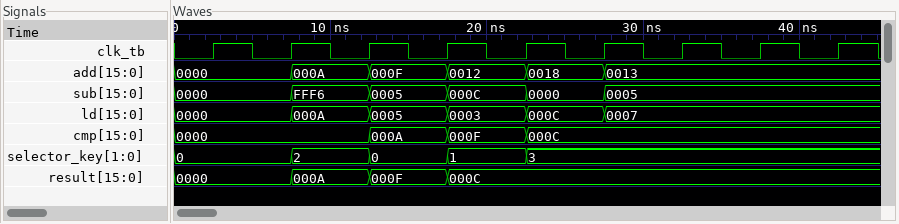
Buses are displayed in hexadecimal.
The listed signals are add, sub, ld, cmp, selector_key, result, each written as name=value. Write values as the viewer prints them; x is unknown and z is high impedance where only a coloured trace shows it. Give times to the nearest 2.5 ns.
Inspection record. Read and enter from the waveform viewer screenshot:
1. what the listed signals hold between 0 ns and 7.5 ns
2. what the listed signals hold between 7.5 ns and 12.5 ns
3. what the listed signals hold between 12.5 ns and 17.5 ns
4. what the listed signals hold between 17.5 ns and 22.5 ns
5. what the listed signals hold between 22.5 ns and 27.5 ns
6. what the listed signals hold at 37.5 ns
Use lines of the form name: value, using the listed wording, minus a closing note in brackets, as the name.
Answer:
what the listed signals hold between 0 ns and 7.5 ns: add=0000, sub=0000, ld=0000, cmp=0000, selector_key=0, result=0000
what the listed signals hold between 7.5 ns and 12.5 ns: add=000A, sub=FFF6, ld=000A, cmp=0000, selector_key=2, result=000A
what the listed signals hold between 12.5 ns and 17.5 ns: add=000F, sub=0005, ld=0005, cmp=000A, selector_key=0, result=000F
what the listed signals hold between 17.5 ns and 22.5 ns: add=0012, sub=000C, ld=0003, cmp=000F, selector_key=1, result=000C
what the listed signals hold between 22.5 ns and 27.5 ns: add=0018, sub=0000, ld=000C, cmp=000C, selector_key=3, result=000C
what the listed signals hold at 37.5 ns: add=0013, sub=0005, ld=0007, cmp=000C, selector_key=3, result=000C
